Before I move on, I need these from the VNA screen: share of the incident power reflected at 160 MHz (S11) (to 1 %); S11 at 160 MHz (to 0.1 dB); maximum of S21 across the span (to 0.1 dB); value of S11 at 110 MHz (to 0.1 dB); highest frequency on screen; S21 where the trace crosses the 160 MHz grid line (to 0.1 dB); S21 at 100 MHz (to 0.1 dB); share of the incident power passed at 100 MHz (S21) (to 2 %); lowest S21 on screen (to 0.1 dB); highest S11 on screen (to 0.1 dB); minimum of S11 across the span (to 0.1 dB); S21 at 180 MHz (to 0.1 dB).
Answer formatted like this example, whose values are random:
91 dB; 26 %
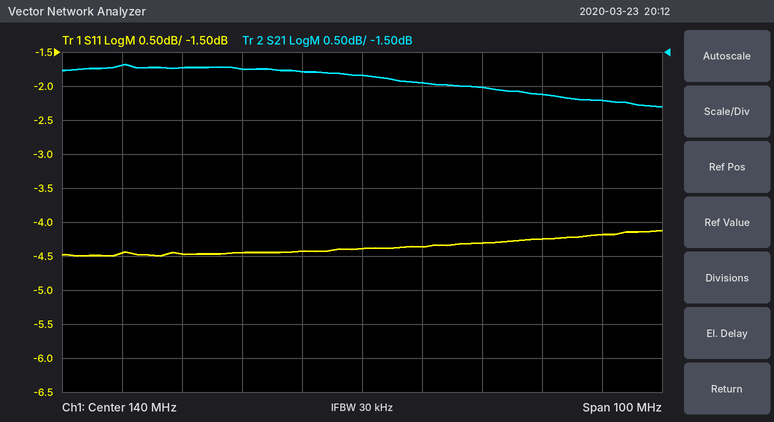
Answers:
37 %; -4.3 dB; -1.7 dB; -4.5 dB; 190 MHz; -2.0 dB; -1.7 dB; 68 %; -2.3 dB; -4.1 dB; -4.5 dB; -2.2 dB
